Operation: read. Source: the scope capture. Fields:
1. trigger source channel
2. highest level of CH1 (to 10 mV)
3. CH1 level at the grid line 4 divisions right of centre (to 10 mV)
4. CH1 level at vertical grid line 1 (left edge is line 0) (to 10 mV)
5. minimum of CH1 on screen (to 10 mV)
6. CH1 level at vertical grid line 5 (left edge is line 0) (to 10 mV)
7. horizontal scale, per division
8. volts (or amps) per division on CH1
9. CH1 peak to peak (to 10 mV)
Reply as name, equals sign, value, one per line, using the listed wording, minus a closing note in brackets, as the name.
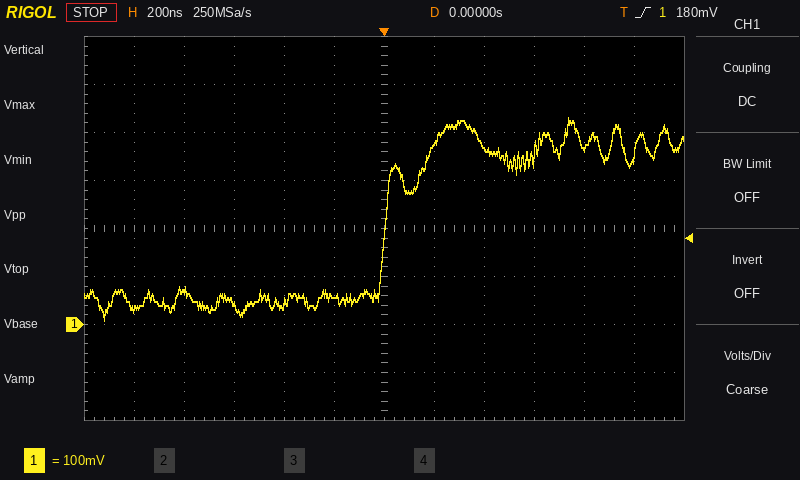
trigger source channel = CH1
highest level of CH1 = 430 mV
CH1 level at the grid line 4 divisions right of centre = 370 mV
CH1 level at vertical grid line 1 (left edge is line 0) = 30 mV
minimum of CH1 on screen = 10 mV
CH1 level at vertical grid line 5 (left edge is line 0) = 60 mV
horizontal scale, per division = 200 ns
volts (or amps) per division on CH1 = 100 mV
CH1 peak to peak = 420 mV
